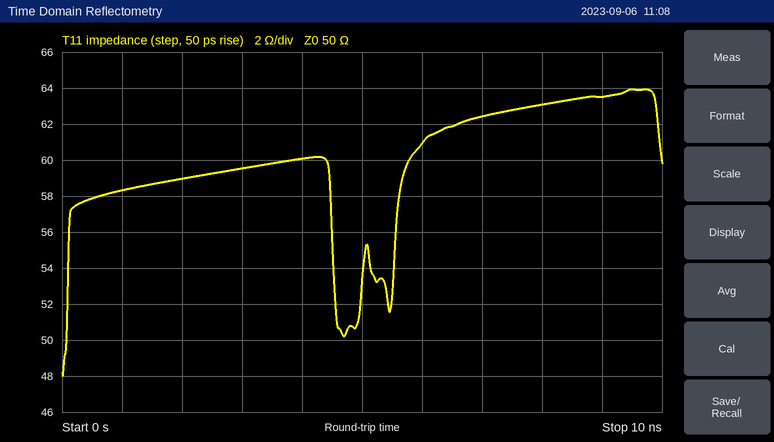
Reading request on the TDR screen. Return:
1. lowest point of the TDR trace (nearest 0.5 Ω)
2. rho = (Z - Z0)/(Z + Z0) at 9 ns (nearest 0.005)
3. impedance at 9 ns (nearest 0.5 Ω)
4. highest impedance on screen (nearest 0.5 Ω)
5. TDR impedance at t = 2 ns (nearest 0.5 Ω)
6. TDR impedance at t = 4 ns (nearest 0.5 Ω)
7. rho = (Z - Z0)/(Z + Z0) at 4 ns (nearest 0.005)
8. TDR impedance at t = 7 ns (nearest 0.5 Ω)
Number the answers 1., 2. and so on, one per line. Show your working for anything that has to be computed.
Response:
1. 48.0 Ω
2. (63.5 − 50)/(63.5 + 50) ≈ +0.119, so +0.120 to the nearest 0.005
3. 63.5 Ω
4. 64.0 Ω
5. 59.0 Ω
6. 60.0 Ω
7. (60 − 50)/(60 + 50) ≈ +0.0909, so +0.090 to the nearest 0.005
8. 62.5 Ω
